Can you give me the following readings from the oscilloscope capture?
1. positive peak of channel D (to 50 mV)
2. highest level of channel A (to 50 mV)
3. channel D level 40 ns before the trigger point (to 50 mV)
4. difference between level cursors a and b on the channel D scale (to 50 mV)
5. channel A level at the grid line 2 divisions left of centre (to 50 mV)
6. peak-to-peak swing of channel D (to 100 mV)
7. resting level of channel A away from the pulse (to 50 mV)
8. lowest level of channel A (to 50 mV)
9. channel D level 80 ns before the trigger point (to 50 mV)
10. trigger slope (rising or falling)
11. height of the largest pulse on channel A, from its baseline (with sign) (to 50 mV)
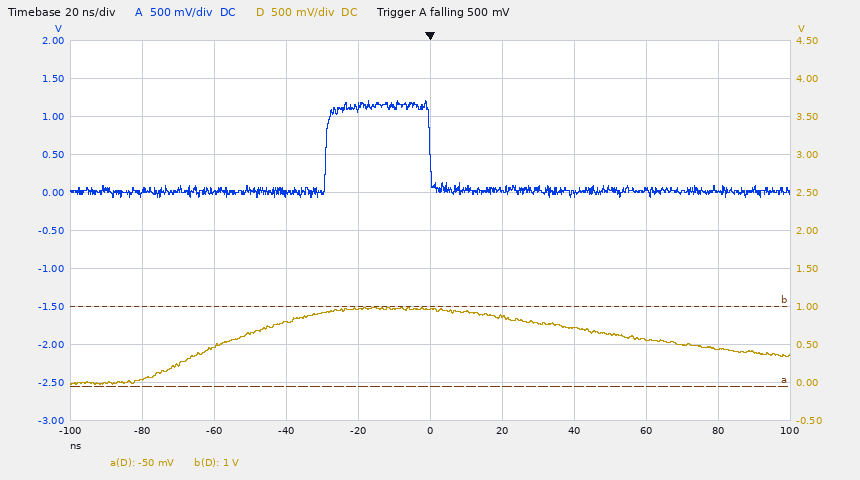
1.00 V
1.20 V
800 mV
1.05 V
0 mV
1.00 V
0 mV
-50 mV
50 mV
falling
+1.20 V
